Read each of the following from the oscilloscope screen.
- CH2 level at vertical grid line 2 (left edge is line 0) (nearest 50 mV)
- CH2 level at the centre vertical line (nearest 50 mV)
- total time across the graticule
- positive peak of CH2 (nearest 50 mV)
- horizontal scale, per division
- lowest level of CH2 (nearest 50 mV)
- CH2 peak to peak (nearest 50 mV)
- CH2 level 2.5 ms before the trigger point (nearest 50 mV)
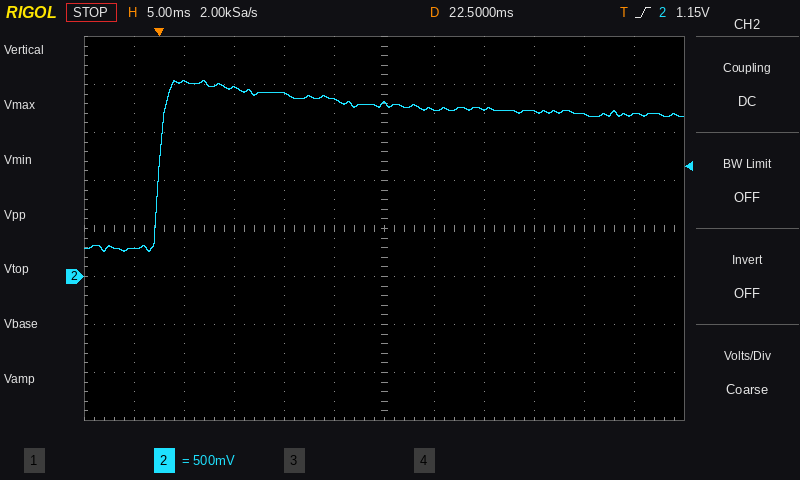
2.05 V
1.80 V
60 ms
2.05 V
5 ms
250 mV
1.80 V
300 mV
